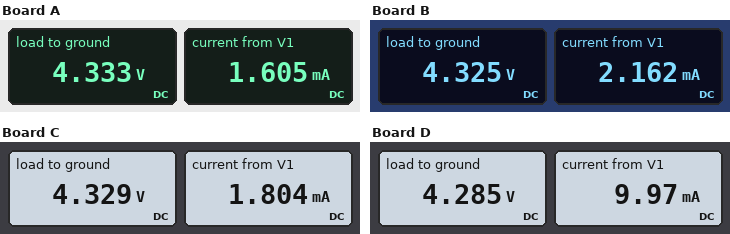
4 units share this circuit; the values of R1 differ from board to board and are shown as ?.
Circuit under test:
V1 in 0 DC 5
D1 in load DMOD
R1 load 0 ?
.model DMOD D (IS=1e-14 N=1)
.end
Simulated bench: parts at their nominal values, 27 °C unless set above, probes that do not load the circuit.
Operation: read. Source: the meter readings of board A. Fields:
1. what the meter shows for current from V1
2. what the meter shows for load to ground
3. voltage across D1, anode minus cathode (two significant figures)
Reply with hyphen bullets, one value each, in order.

- 1.605 mA
- 4.333 V
- 670 mV
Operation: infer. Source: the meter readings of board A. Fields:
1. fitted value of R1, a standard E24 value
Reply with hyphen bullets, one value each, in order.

- 2.7 kΩ
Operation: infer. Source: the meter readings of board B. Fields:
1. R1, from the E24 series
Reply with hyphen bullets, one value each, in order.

- 2 kΩ
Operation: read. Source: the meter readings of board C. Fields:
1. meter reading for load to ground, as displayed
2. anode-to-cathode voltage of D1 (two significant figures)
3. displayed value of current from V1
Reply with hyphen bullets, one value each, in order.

- 4.329 V
- 670 mV
- 1.804 mA
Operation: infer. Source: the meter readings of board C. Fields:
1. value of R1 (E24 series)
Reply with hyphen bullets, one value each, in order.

- 2.4 kΩ
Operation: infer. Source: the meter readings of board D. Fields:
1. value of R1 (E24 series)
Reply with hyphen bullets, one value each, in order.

- 430 Ω
